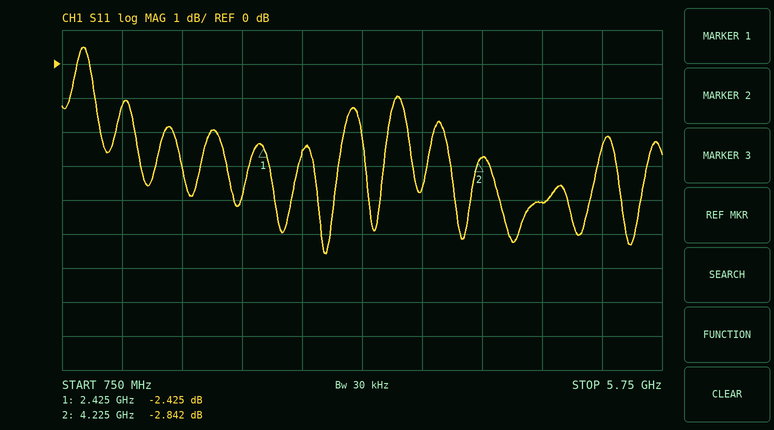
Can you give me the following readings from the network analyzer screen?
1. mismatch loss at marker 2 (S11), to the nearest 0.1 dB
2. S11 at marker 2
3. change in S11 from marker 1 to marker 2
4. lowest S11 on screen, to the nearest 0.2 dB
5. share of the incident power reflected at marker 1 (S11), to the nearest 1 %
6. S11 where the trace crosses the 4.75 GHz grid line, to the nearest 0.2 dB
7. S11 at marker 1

3.2 dB
-2.842 dB
-0.417 dB
-5.6 dB
57 %
-4.0 dB
-2.425 dB
